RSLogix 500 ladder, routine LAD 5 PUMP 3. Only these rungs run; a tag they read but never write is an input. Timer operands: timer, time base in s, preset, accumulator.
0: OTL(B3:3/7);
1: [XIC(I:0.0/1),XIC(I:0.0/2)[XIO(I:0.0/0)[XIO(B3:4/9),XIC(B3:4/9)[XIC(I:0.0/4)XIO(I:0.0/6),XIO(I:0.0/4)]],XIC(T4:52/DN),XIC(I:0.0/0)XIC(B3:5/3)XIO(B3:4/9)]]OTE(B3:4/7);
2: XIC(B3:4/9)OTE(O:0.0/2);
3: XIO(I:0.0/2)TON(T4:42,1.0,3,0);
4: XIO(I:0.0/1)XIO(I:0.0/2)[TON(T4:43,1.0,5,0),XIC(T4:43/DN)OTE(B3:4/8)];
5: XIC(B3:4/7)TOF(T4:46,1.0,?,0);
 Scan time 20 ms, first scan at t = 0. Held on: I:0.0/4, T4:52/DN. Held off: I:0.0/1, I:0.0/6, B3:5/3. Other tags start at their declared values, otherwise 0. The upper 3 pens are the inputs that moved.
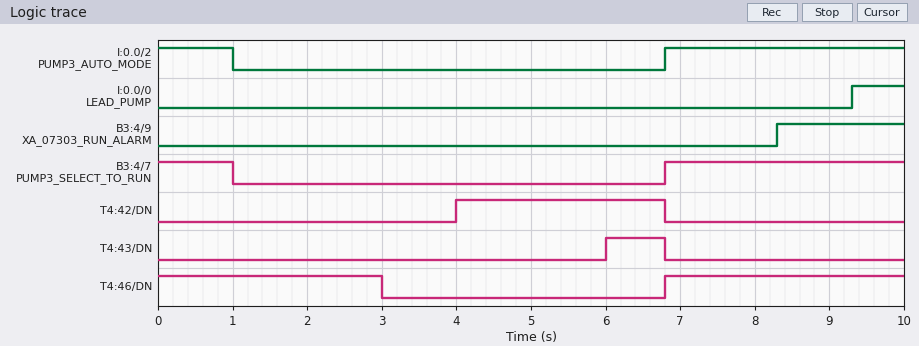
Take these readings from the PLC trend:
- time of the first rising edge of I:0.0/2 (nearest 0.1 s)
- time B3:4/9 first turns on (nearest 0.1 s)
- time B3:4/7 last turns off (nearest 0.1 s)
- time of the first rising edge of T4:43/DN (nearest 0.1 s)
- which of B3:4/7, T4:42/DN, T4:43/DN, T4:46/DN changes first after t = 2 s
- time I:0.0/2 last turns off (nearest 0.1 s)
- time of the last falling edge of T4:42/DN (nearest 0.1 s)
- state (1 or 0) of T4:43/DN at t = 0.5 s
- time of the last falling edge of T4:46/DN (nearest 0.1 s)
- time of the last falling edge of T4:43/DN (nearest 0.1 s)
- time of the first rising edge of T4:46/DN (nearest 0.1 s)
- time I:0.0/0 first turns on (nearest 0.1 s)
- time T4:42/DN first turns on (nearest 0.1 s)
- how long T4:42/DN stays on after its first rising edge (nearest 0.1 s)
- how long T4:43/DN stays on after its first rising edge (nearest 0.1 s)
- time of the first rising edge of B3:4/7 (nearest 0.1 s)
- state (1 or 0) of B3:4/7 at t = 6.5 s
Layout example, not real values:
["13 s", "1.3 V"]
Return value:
["6.8 s", "8.3 s", "1.0 s", "6.0 s", "T4:46/DN", "1.0 s", "6.8 s", "0", "3.0 s", "6.8 s", "6.8 s", "9.3 s", "4.0 s", "2.8 s", "0.8 s", "6.8 s", "0"]
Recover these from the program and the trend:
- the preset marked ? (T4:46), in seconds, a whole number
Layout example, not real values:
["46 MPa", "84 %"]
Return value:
["2 s"]
